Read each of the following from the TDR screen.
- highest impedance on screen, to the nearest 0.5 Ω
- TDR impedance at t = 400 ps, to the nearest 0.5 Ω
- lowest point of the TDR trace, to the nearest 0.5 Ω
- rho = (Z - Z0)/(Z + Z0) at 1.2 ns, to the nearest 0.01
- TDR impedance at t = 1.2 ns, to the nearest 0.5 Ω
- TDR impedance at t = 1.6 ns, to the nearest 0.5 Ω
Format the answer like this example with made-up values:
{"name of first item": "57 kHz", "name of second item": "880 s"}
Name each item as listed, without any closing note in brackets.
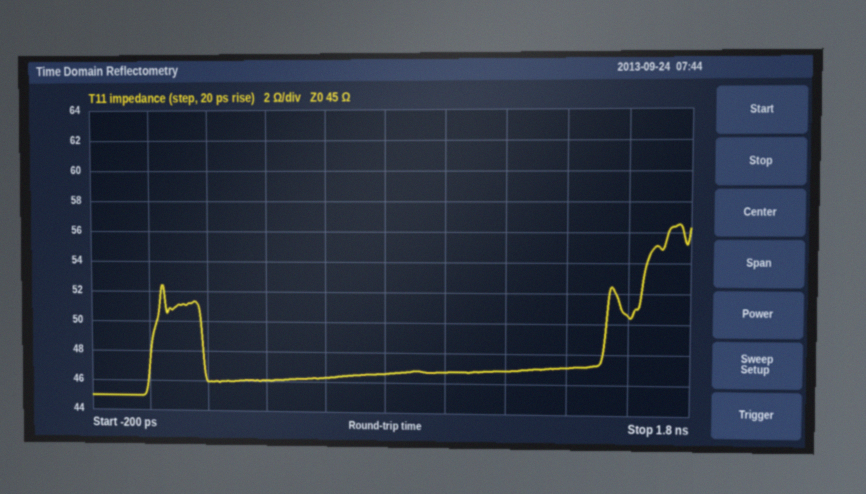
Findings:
{"highest impedance on screen, to the nearest 0.5 Ω": "56.5 Ω", "TDR impedance at t = 400 ps, to the nearest 0.5 Ω": "46.0 Ω", "lowest point of the TDR trace, to the nearest 0.5 Ω": "45.0 Ω", "rho = (Z - Z0)/(Z + Z0) at 1.2 ns, to the nearest 0.01": "+0.02", "TDR impedance at t = 1.2 ns, to the nearest 0.5 Ω": "47.0 Ω", "TDR impedance at t = 1.6 ns, to the nearest 0.5 Ω": "50.5 Ω"}
